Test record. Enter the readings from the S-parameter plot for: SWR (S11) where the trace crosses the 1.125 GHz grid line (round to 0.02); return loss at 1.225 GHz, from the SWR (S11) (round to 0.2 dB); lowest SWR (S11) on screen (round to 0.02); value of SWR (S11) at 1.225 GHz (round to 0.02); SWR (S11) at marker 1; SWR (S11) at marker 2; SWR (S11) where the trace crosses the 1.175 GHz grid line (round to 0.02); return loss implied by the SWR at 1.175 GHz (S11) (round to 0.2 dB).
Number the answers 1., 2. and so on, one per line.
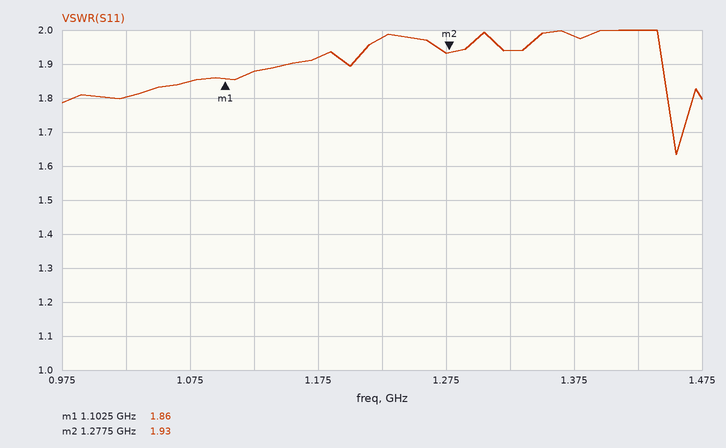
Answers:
1. 1.88
2. 9.6 dB
3. 1.64
4. 1.98
5. 1.86
6. 1.93
7. 1.92
8. 10.0 dB
